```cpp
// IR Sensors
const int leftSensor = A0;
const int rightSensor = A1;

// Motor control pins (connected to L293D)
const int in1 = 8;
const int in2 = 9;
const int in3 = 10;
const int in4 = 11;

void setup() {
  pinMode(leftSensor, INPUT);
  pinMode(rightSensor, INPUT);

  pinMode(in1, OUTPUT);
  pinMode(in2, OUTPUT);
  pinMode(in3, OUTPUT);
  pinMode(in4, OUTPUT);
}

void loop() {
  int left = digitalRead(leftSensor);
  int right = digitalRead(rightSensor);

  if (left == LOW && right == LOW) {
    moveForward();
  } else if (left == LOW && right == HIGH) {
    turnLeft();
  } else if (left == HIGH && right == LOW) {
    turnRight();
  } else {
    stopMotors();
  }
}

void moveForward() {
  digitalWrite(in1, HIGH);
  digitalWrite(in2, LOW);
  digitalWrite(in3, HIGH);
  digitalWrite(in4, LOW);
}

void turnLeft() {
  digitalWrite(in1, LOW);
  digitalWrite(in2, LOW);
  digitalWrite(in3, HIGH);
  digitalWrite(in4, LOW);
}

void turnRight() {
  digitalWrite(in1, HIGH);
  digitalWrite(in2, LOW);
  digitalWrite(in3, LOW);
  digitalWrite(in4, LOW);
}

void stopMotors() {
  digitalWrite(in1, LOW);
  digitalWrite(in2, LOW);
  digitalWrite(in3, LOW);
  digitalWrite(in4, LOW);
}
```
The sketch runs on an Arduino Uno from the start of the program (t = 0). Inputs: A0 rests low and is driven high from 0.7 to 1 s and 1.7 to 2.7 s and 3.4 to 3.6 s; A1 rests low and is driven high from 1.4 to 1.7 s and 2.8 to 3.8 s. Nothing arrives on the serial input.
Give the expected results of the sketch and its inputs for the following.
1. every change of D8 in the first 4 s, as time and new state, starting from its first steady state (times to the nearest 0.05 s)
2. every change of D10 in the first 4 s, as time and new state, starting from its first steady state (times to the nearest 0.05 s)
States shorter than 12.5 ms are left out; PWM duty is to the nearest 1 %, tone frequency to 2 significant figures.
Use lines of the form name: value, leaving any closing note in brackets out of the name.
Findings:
every change of D8 in the first 4 s, as time and new state, starting from its first steady state: 0 s high; 1.4 s low; 1.7 s high; 2.8 s low; 3.8 s high
every change of D10 in the first 4 s, as time and new state, starting from its first steady state: 0 s high; 0.7 s low; 1 s high; 1.7 s low; 2.7 s high; 3.4 s low; 3.6 s high
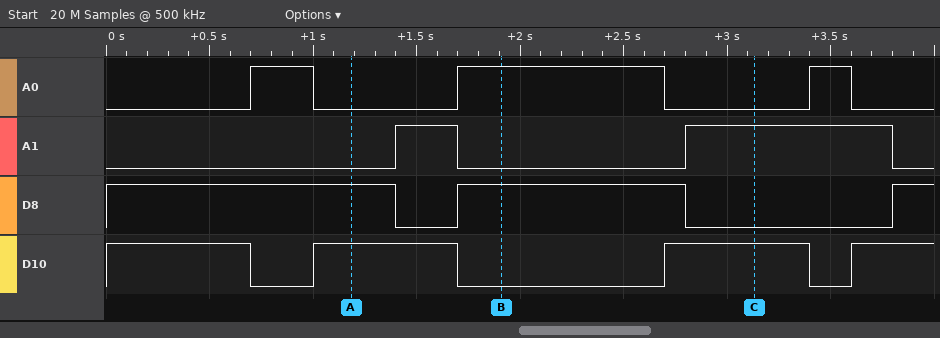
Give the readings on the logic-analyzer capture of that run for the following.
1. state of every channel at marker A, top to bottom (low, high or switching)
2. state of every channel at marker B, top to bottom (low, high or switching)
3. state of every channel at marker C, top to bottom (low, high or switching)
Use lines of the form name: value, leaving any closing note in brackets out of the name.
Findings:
state of every channel at marker A, top to bottom: A0 low, A1 low, D8 high, D10 high
state of every channel at marker B, top to bottom: A0 high, A1 low, D8 high, D10 low
state of every channel at marker C, top to bottom: A0 low, A1 high, D8 low, D10 high
